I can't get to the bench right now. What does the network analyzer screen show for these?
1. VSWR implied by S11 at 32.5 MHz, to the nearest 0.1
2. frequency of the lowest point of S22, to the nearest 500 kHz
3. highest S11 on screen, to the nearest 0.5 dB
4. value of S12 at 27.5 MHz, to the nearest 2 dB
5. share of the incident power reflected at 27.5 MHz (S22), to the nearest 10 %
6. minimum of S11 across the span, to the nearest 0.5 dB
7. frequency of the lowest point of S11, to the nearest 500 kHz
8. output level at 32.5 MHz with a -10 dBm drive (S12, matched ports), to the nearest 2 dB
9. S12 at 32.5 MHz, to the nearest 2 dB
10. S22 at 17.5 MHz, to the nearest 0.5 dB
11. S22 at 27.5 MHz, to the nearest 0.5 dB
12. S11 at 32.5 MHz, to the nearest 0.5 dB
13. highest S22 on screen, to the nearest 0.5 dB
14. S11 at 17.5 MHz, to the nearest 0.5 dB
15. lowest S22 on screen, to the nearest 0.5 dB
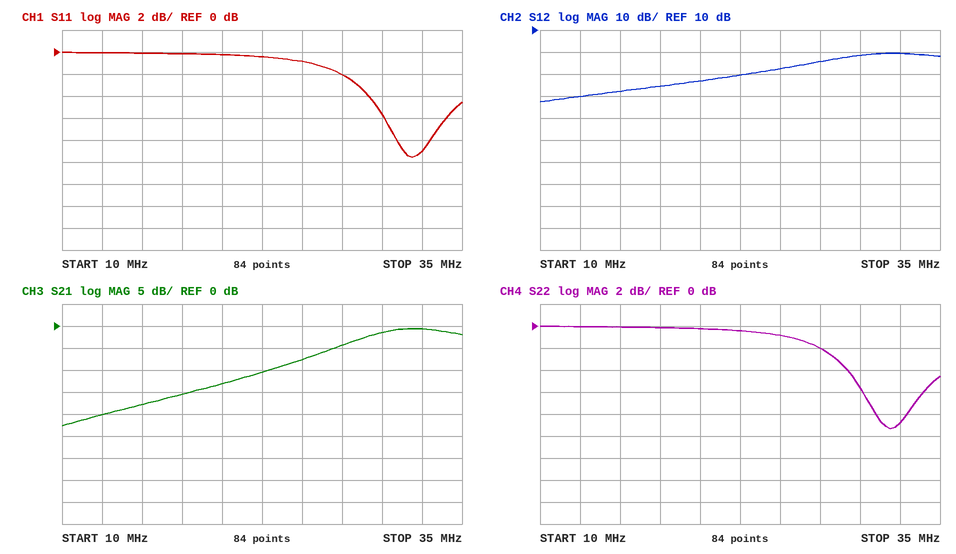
2.1
32.0 MHz
0.0 dB
-4 dB
60 %
-9.5 dB
32.0 MHz
-10 dBm
0 dB
0.0 dB
-2.0 dB
-9.0 dB
0.0 dB
0.0 dB
-9.5 dB
